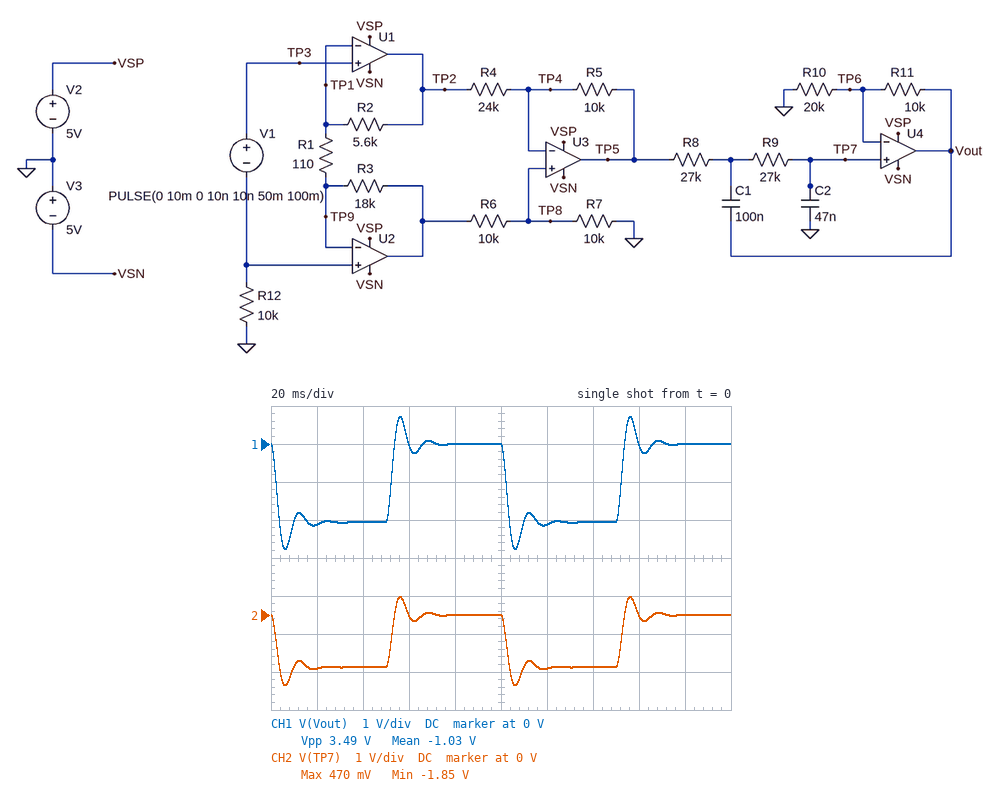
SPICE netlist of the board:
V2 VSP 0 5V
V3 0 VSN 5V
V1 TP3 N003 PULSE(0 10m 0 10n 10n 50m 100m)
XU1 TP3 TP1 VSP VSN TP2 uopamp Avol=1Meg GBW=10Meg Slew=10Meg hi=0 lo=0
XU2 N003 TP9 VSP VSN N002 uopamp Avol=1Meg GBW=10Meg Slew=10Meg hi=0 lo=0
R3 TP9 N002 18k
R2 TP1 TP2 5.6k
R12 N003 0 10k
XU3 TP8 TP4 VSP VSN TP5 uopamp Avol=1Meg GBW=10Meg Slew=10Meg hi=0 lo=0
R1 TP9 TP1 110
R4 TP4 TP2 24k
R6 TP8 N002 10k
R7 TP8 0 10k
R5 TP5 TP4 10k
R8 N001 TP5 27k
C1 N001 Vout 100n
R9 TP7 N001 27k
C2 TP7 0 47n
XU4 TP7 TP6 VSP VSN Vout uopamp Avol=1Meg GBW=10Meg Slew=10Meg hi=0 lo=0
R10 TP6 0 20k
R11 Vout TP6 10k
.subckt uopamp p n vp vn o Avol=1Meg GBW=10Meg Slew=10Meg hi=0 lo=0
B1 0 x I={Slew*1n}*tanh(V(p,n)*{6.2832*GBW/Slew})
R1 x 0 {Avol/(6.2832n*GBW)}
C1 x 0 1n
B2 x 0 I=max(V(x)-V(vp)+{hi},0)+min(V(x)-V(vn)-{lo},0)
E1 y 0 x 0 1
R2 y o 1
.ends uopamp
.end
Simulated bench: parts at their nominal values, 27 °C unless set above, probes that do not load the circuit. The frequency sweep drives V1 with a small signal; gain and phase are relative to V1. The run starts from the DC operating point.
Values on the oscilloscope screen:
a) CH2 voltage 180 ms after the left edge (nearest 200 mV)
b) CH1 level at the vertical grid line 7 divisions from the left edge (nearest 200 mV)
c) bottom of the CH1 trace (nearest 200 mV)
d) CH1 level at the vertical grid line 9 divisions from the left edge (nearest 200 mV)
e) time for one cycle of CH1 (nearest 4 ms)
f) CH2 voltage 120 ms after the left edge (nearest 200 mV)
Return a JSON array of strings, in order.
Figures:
["0 V", "-2.0 V", "-2.8 V", "0 V", "100 ms", "-1.4 V"]
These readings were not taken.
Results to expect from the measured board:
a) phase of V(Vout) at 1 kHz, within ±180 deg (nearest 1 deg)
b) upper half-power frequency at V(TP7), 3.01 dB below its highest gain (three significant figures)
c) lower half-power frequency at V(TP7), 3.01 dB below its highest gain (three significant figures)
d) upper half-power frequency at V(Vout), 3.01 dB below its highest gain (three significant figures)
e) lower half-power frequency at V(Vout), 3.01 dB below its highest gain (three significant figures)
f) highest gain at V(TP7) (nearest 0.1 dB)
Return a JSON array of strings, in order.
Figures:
["2 deg", "102 Hz", "37.1 Hz", "102 Hz", "37.1 Hz", "47.1 dB"]
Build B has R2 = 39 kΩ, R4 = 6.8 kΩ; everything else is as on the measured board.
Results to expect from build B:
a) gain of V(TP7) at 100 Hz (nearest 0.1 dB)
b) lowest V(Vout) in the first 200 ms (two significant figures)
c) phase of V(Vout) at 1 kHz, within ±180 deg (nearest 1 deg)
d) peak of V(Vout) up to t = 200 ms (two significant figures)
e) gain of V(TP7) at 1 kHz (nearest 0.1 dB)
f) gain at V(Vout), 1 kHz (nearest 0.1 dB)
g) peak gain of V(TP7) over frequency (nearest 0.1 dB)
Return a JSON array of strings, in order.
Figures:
["58.9 dB", "-5.0 V", "0 deg", "1.9 V", "14.6 dB", "18.1 dB", "61.5 dB"]
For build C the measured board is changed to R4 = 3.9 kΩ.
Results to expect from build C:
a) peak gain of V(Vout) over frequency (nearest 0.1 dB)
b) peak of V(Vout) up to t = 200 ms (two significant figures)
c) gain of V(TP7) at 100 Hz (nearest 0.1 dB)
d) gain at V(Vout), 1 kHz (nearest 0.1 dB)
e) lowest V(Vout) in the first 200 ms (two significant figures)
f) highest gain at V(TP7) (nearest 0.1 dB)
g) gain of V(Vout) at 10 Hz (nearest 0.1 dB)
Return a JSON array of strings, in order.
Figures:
["60.4 dB", "1.9 V", "54.2 dB", "13.5 dB", "-5.0 V", "56.9 dB", "56.2 dB"]
